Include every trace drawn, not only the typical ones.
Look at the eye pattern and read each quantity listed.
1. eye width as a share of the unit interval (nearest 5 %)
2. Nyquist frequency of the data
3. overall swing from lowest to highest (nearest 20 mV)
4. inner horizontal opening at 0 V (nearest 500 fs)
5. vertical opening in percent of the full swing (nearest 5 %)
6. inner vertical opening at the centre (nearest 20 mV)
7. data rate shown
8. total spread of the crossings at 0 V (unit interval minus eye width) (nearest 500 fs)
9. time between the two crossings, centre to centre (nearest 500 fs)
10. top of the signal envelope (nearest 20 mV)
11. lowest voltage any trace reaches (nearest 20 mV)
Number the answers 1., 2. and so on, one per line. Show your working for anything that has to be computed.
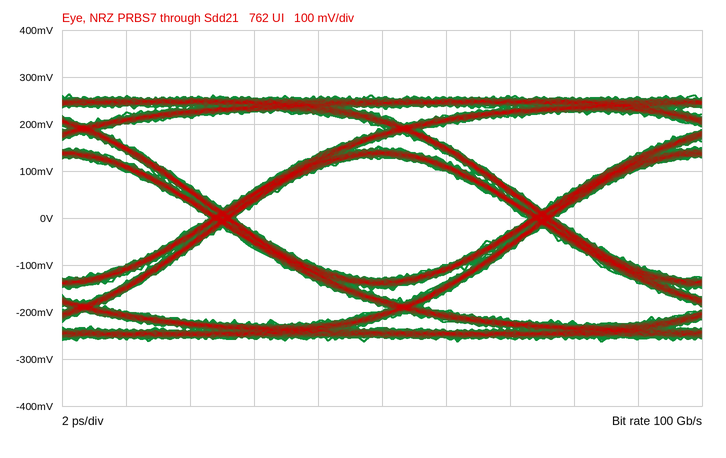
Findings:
1. 9.0 ps / 10.0 ps ≈ 90 %
2. 50 GHz
3. 520 mV
4. 9.0 ps
5. 260 mV / 520 mV ≈ 50 %
6. 260 mV
7. 100 Gb/s
8. 1.0 ps
9. 10.0 ps
10. 260 mV
11. -260 mV
